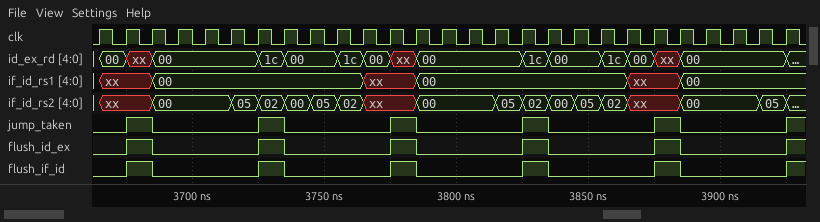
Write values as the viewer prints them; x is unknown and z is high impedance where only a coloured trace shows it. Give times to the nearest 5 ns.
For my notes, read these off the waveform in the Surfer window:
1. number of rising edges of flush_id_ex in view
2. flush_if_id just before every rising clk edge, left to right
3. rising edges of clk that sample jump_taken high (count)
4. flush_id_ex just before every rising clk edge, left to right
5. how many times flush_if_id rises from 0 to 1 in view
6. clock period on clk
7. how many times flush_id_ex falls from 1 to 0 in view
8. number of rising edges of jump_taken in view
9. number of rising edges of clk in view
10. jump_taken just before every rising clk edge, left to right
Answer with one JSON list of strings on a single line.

["6", "0 0 1 0 0 0 0 1 0 0 0 0 1 0 0 0 0 1 0 0 0 0 1 0 0 0 0", "5", "0 0 1 0 0 0 0 1 0 0 0 0 1 0 0 0 0 1 0 0 0 0 1 0 0 0 0", "6", "10 ns", "5", "6", "27", "0 0 1 0 0 0 0 1 0 0 0 0 1 0 0 0 0 1 0 0 0 0 1 0 0 0 0"]
